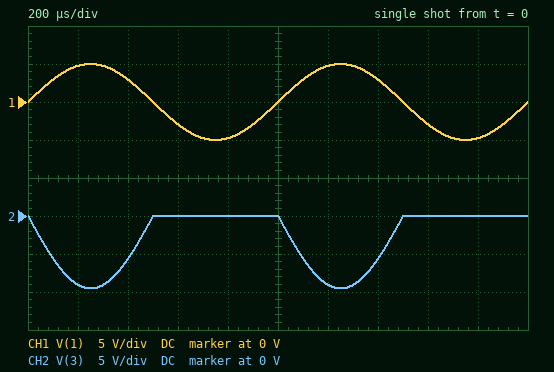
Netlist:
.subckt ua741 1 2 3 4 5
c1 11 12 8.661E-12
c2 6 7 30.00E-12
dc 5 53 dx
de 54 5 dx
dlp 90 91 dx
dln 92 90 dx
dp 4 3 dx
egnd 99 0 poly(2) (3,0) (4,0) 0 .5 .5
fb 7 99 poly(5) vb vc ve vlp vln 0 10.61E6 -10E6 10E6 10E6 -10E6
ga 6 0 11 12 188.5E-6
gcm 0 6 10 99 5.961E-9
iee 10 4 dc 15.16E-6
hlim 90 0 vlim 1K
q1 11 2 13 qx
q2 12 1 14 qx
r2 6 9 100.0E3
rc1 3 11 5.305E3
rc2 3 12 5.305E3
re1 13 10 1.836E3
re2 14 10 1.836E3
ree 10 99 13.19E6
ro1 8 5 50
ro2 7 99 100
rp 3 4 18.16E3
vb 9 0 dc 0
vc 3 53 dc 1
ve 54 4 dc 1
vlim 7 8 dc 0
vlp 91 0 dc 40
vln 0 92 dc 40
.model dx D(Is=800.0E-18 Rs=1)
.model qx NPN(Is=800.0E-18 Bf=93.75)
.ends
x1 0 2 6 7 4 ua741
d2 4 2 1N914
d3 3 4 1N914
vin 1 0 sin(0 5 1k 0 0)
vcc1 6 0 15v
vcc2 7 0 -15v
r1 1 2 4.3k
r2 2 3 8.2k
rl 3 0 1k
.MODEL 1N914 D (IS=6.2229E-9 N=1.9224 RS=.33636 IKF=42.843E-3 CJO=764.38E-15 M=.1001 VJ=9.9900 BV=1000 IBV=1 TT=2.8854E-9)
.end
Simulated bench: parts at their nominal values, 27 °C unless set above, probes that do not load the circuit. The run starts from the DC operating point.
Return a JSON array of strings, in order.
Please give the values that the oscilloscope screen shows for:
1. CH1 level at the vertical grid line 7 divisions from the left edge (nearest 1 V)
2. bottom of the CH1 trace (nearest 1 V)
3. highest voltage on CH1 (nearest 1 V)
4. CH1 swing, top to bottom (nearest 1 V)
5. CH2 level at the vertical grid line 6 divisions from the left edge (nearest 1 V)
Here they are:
["3 V", "-5 V", "5 V", "10 V", "-9 V"]
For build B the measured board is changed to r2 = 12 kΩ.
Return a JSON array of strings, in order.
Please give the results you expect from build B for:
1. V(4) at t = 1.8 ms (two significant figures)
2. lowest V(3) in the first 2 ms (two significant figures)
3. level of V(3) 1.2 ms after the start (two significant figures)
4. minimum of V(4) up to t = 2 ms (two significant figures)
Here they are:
["610 mV", "-14 V", "-13 V", "-15 V"]
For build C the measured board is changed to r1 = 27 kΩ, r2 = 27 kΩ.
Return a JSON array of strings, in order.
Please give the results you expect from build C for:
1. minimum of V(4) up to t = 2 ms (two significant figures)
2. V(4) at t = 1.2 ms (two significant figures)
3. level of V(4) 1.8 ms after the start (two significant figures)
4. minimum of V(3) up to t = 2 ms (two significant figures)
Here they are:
["-5.7 V", "-5.4 V", "510 mV", "-5.0 V"]
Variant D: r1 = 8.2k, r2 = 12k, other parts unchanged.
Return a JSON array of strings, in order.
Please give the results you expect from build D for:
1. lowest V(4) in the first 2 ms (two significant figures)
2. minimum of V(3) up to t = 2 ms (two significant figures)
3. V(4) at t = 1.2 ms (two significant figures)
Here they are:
["-8.0 V", "-7.3 V", "-7.7 V"]
